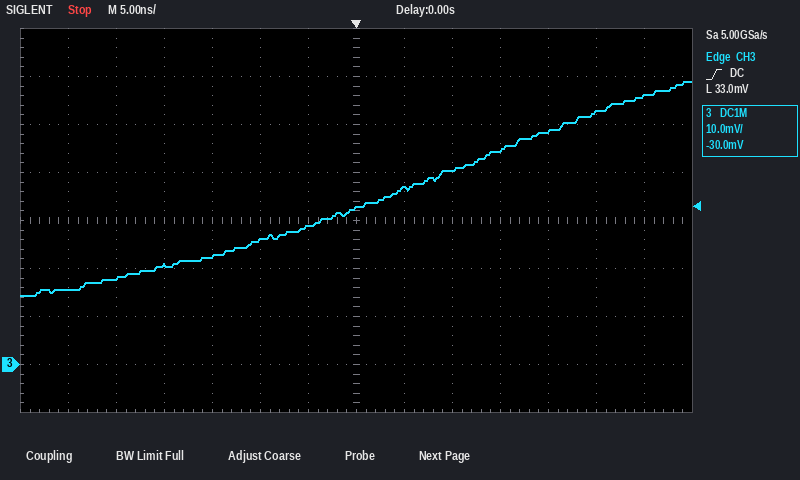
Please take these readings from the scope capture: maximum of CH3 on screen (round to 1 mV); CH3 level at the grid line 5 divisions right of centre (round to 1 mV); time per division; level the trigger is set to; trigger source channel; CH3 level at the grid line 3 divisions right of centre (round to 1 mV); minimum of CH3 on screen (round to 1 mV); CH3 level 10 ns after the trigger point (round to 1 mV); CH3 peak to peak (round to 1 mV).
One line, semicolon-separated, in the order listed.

59 mV; 53 mV; 5 ns; 33.0 mV; CH3; 45 mV; 14 mV; 40 mV; 45 mV
